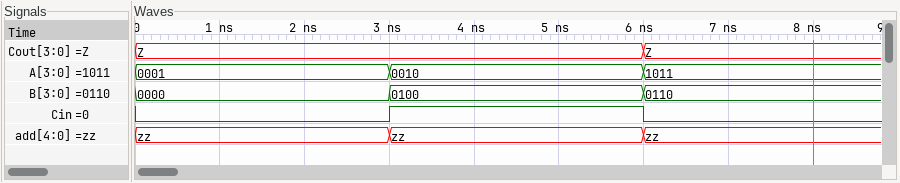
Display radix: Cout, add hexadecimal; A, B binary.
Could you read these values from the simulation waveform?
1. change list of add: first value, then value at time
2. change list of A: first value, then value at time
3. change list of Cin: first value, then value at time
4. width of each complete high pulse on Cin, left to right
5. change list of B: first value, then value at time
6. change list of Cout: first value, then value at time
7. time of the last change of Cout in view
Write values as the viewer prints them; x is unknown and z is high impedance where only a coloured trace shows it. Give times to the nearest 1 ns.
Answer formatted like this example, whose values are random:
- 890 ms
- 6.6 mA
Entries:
- zz, zz at 3 ns, zz at 6 ns
- 0001, 0010 at 3 ns, 1011 at 6 ns
- 0, 1 at 3 ns, 0 at 6 ns
- 3 ns
- 0000, 0100 at 3 ns, 0110 at 6 ns
- Z, Z at 6 ns
- 6 ns
